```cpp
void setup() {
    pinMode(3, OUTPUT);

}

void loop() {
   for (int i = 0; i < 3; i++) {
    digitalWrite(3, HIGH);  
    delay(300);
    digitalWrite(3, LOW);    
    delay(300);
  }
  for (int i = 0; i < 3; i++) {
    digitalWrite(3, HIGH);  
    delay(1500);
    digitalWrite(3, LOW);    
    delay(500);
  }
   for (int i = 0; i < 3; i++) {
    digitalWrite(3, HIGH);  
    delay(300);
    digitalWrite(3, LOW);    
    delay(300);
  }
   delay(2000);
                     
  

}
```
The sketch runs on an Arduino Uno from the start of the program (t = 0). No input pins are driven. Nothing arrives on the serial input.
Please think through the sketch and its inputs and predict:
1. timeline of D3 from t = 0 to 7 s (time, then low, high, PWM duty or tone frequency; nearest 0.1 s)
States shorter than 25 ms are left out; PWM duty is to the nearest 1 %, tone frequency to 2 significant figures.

0 s high; 0.3 s low; 0.6 s high; 0.9 s low; 1.2 s high; 1.5 s low; 1.8 s high; 3.3 s low; 3.8 s high; 5.3 s low; 5.8 s high
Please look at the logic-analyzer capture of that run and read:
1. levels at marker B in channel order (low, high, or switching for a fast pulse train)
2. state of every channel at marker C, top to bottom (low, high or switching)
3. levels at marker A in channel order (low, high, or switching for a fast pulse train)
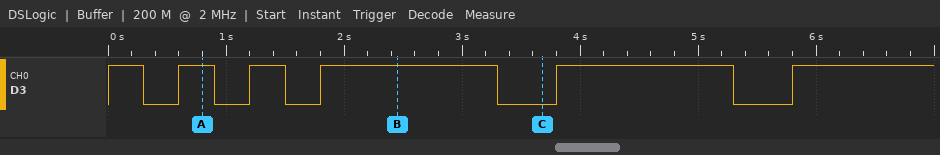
D3 high
D3 low
D3 high
